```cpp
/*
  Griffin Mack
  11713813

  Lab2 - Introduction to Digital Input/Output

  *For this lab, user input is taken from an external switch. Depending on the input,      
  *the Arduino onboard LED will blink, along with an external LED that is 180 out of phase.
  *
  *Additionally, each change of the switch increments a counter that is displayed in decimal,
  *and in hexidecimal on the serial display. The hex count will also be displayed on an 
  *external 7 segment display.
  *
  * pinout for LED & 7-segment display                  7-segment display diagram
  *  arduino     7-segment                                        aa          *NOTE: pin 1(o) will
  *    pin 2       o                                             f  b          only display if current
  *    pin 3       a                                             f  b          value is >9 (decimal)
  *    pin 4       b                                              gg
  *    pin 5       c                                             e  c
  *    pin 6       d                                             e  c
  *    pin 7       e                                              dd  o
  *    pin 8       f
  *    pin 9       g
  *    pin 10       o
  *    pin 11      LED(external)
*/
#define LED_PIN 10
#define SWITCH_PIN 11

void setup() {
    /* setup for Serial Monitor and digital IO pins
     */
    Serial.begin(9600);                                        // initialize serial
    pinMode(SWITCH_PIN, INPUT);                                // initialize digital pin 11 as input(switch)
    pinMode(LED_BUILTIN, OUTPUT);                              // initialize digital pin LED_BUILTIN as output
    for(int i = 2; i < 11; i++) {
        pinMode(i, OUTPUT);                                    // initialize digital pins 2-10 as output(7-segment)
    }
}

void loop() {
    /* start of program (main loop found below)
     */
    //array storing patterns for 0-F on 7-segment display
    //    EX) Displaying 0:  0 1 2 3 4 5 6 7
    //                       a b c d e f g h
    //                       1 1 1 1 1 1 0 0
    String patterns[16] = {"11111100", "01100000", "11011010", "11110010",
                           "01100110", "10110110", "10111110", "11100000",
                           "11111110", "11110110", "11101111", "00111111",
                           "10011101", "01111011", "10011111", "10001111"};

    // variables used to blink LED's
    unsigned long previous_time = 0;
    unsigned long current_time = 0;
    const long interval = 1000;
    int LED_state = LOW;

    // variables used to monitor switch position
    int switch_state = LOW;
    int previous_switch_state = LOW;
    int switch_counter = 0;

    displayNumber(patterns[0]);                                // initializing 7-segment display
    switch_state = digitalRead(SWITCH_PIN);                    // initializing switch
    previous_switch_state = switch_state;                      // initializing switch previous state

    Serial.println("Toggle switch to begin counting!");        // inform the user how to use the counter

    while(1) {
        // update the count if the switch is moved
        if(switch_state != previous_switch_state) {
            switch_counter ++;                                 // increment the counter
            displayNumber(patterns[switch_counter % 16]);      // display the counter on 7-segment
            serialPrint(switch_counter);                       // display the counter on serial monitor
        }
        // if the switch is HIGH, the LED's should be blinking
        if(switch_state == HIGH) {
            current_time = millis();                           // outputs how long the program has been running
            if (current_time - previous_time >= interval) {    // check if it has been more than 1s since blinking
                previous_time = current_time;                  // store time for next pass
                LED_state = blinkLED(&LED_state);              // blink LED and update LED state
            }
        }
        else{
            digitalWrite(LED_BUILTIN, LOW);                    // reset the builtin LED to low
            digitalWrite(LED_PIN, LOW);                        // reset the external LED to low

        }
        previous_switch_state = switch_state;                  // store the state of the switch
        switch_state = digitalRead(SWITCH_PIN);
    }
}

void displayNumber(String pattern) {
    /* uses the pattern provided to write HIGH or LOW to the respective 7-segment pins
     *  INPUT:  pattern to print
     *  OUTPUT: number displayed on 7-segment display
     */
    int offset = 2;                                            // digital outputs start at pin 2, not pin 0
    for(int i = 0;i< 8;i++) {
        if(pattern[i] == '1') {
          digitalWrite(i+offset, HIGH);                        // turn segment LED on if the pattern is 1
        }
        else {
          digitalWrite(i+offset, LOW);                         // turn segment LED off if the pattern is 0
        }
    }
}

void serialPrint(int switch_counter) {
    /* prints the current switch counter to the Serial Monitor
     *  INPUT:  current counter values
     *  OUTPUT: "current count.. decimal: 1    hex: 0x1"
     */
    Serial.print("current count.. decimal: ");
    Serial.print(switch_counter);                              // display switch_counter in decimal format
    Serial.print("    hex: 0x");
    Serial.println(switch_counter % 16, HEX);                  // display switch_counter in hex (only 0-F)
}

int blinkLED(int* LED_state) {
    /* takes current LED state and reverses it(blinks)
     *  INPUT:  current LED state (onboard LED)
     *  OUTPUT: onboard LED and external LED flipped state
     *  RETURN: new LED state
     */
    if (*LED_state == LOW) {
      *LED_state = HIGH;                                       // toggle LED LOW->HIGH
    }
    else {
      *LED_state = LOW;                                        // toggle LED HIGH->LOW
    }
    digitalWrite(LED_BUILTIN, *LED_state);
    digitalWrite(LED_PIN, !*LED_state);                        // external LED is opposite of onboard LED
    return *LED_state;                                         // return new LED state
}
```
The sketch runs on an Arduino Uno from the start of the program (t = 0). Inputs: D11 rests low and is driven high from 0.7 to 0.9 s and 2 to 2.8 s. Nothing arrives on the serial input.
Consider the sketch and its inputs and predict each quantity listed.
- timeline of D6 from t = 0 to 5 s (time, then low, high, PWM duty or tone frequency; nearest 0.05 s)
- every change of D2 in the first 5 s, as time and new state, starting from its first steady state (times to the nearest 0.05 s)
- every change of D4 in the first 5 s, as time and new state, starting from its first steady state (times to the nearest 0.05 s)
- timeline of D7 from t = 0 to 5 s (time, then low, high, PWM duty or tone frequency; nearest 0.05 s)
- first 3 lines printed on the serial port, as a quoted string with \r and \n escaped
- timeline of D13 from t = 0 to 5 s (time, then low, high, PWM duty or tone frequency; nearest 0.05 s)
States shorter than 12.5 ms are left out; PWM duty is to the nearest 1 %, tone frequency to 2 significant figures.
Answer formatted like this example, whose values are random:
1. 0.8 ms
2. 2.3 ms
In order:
1. 0 s high; 0.7 s low; 0.9 s high; 2 s low
2. 0 s high; 0.7 s low; 0.9 s high; 2.8 s low
3. 0 s high; 0.9 s low; 2 s high
4. 0 s high; 0.7 s low; 2.8 s high
5. "Toggle switch to begin counting!\r\ncurrent count.. decimal: 1    hex: 0x1\r\ncurrent count.. decimal: 2    hex: 0x2\r\n"
6. 0 s low; 2 s high; 2.8 s low
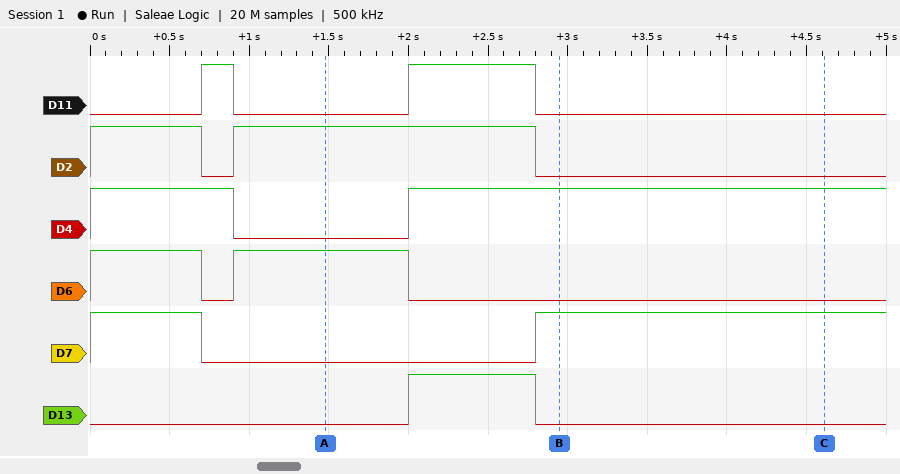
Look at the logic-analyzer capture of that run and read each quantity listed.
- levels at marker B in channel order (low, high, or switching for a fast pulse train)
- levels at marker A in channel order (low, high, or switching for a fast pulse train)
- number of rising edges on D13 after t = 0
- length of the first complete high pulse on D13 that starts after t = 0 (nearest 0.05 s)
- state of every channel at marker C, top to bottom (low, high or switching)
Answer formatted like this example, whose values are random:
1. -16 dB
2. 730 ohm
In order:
1. D11 low, D2 low, D4 high, D6 low, D7 high, D13 low
2. D11 low, D2 high, D4 low, D6 high, D7 low, D13 low
3. 1
4. 0.80 s
5. D11 low, D2 low, D4 high, D6 low, D7 high, D13 low
